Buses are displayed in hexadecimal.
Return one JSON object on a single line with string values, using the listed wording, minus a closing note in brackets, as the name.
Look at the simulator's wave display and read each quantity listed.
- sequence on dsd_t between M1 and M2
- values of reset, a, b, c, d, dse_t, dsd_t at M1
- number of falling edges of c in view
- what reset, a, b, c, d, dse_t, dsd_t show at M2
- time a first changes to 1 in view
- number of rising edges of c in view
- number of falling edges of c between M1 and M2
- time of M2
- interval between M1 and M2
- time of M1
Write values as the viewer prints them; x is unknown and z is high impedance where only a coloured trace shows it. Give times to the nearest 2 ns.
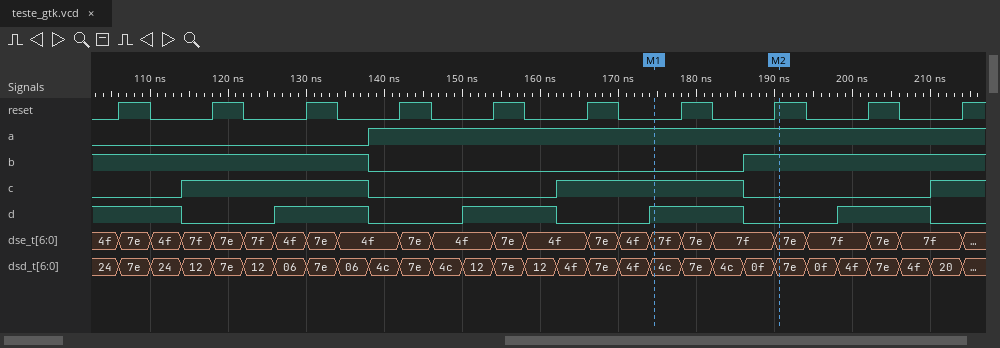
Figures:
{"sequence on dsd_t between M1 and M2": "4c, 7e, 4c, 0f, 7e", "values of reset, a, b, c, d, dse_t, dsd_t at M1": "reset=0, a=1, b=0, c=1, d=1, dse_t=7f, dsd_t=4c", "number of falling edges of c in view": "2", "what reset, a, b, c, d, dse_t, dsd_t show at M2": "reset=1, a=1, b=1, c=0, d=0, dse_t=7e, dsd_t=7e", "time a first changes to 1 in view": "138 ns", "number of rising edges of c in view": "3", "number of falling edges of c between M1 and M2": "1", "time of M2": "190 ns", "interval between M1 and M2": "16 ns", "time of M1": "174 ns"}
